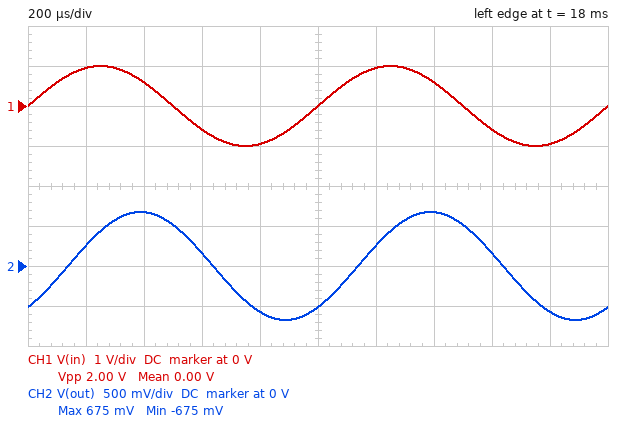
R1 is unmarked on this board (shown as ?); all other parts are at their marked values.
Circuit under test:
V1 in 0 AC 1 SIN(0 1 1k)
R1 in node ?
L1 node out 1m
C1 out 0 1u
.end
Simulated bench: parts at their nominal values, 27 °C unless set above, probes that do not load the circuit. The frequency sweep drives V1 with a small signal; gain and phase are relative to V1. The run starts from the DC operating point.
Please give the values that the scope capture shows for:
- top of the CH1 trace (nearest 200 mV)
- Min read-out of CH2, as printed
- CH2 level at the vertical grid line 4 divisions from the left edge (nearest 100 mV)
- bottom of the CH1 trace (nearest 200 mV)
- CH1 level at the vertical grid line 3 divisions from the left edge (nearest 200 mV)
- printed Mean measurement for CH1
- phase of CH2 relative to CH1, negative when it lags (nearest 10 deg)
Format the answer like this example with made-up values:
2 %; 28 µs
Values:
1.0 V; -675 mV; -600 mV; -1.0 V; -600 mV; 0.00 V; -50 deg
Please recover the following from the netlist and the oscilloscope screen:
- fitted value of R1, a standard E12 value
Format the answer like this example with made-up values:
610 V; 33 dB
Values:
180 Ω
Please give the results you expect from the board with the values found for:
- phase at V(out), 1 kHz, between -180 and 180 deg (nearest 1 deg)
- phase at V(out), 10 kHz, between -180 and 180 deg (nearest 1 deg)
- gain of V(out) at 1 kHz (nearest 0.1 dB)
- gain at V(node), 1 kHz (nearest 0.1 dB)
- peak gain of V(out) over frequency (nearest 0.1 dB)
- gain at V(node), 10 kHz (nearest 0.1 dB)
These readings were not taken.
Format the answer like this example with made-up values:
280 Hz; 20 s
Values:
-50 deg; -105 deg; -3.4 dB; -3.8 dB; 0 dB; -12.0 dB
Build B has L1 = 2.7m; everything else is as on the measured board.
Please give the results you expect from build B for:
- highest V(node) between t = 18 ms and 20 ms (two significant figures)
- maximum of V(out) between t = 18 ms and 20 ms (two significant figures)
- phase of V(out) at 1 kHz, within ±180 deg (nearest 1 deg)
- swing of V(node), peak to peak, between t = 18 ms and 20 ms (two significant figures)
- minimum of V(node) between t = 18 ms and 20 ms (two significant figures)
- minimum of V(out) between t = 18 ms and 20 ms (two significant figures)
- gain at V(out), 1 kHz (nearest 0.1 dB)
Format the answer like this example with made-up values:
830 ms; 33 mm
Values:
620 mV; 690 mV; -52 deg; 1.2 V; -620 mV; -690 mV; -3.2 dB
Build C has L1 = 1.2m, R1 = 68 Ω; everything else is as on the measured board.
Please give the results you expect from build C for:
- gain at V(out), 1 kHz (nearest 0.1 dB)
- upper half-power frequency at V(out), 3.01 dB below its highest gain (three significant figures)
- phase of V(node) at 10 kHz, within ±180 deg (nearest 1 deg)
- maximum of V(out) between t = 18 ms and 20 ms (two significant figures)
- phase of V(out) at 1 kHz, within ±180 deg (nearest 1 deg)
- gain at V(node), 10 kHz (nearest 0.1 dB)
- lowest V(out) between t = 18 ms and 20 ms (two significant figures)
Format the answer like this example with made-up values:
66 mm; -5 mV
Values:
-0.4 dB; 3.04 kHz; 49 deg; 960 mV; -24 deg; -3.6 dB; -960 mV
